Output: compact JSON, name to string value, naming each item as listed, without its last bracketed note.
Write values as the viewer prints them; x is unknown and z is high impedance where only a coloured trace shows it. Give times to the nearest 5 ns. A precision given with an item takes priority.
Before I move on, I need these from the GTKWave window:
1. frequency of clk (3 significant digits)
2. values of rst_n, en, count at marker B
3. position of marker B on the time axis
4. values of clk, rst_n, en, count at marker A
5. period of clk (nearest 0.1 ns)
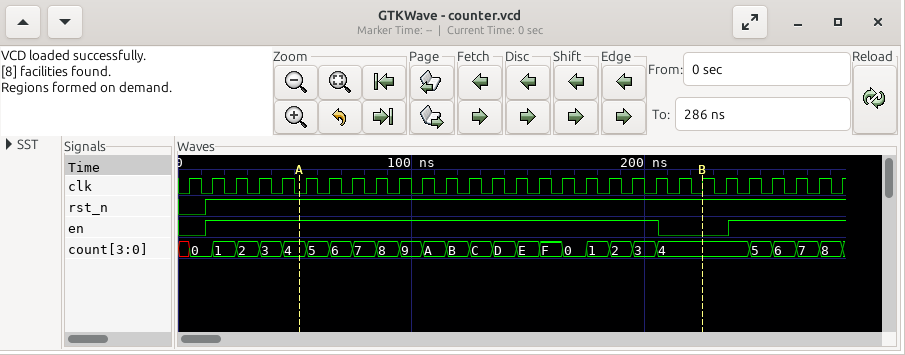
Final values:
{"frequency of clk": "100 MHz", "values of rst_n, en, count at marker B": "rst_n=1, en=0, count=4", "position of marker B on the time axis": "225 ns", "values of clk, rst_n, en, count at marker A": "clk=0, rst_n=1, en=1, count=4", "period of clk": "10 ns"}
